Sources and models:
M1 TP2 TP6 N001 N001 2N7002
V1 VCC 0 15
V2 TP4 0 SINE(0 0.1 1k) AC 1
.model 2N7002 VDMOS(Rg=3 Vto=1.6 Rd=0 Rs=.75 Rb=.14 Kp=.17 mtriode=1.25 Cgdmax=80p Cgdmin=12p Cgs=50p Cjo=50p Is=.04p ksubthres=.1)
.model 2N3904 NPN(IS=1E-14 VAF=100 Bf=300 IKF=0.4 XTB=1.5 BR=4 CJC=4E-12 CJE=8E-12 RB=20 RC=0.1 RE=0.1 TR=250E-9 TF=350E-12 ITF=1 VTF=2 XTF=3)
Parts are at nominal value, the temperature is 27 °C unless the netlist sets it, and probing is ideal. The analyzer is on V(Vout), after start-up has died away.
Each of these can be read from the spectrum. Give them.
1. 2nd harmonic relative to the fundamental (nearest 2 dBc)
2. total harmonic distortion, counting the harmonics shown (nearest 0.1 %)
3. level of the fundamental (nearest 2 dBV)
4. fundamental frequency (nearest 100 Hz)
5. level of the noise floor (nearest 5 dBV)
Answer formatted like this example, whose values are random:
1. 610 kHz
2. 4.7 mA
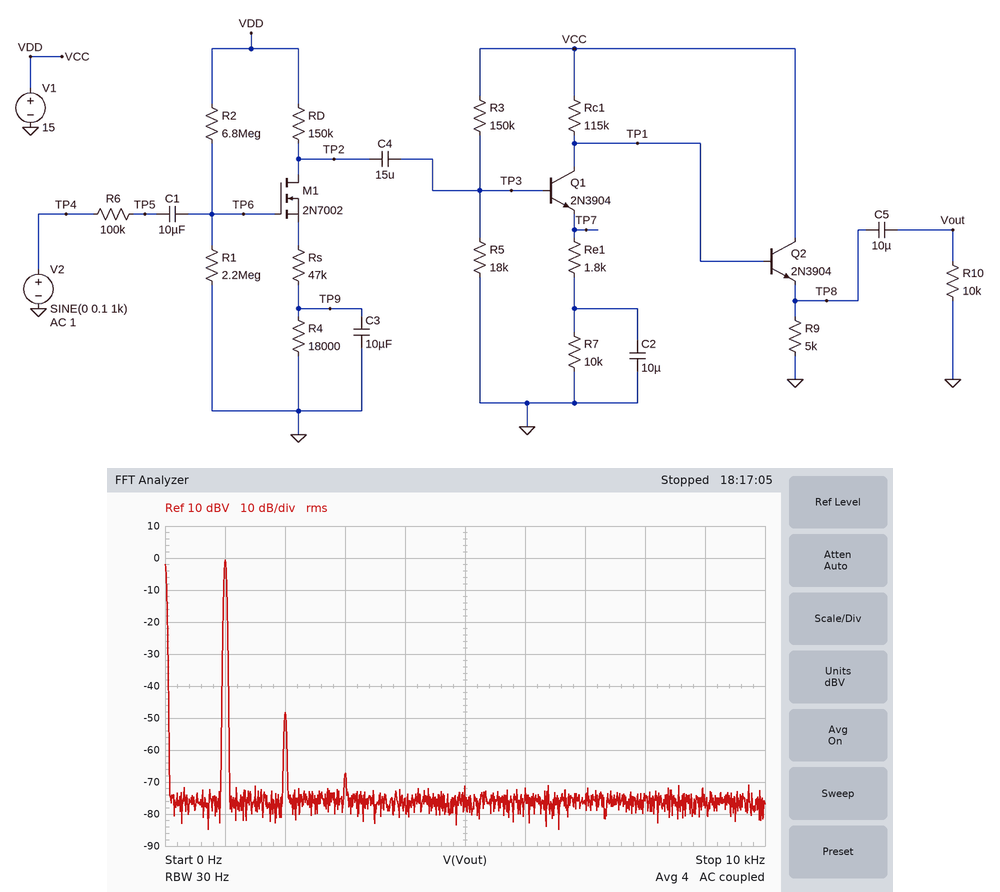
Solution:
1. -48 dBc
2. 0.4 %
3. 0 dBV
4. 1.0 kHz
5. -75 dBV
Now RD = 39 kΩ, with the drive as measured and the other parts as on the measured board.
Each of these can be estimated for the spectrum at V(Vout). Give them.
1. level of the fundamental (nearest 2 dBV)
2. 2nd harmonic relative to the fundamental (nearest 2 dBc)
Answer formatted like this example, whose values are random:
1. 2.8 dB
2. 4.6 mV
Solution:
1. -2 dBV
2. -50 dBc
